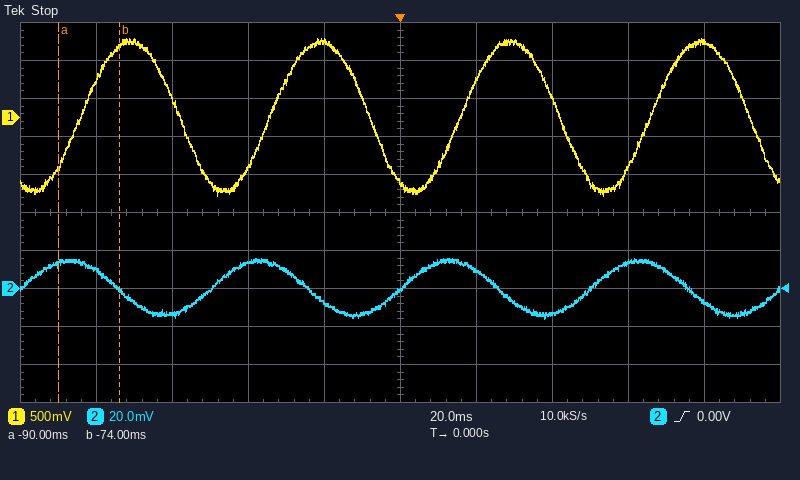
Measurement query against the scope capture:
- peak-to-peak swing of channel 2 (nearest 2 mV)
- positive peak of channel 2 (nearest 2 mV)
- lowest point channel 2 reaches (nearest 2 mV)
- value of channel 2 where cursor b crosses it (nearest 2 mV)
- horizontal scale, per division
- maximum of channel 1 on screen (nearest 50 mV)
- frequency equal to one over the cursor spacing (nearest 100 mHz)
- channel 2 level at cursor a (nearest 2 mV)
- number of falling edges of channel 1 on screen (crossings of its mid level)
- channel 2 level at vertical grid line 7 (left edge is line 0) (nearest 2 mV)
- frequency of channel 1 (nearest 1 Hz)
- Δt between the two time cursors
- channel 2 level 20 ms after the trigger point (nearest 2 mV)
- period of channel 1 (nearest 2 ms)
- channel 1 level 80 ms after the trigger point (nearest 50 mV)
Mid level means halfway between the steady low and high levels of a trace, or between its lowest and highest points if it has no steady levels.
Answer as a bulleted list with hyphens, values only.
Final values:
- 32 mV
- 16 mV
- -16 mV
- 0 mV
- 20 ms
- 1.05 V
- 62.5 Hz
- 14 mV
- 4
- -14 mV
- 20 Hz
- 16 ms
- 10 mV
- 50 ms
- 1.00 V
